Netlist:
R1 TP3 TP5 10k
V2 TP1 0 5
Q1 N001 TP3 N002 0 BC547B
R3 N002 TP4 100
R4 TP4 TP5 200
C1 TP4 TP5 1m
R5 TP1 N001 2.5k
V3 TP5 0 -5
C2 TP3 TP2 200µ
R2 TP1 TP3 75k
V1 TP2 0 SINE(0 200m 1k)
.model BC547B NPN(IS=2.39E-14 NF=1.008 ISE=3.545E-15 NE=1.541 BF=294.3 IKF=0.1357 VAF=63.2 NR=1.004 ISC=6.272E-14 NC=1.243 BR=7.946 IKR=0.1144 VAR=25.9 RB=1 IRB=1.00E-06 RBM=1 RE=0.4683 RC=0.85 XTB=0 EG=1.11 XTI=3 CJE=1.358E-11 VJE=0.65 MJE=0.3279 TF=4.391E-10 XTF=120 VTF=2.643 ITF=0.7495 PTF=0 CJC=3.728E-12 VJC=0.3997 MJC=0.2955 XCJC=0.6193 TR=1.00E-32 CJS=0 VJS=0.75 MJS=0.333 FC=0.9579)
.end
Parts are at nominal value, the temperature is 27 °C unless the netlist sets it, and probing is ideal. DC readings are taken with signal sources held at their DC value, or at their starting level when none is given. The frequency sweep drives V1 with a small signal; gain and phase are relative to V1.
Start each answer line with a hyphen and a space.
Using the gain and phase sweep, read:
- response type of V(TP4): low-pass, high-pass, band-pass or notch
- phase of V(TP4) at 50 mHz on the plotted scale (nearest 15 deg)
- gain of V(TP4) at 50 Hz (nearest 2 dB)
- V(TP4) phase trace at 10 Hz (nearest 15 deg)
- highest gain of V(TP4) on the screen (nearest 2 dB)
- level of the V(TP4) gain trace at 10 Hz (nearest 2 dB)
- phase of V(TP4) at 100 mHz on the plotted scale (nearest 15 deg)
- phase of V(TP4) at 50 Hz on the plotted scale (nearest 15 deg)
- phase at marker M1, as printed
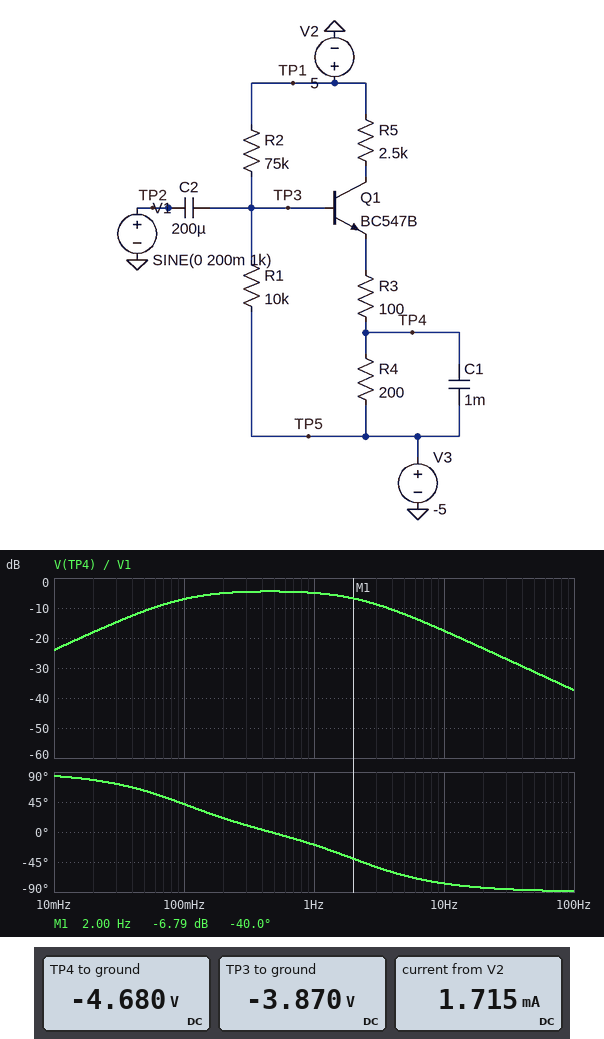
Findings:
- band-pass
- 60 deg
- -32 dB
- -75 deg
- -4 dB
- -18 dB
- 45 deg
- -90 deg
- -40.0 deg
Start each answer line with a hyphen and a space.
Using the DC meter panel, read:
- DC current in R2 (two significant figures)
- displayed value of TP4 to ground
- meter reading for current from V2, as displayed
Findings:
- 120 µA
- -4.680 V
- 1.715 mA
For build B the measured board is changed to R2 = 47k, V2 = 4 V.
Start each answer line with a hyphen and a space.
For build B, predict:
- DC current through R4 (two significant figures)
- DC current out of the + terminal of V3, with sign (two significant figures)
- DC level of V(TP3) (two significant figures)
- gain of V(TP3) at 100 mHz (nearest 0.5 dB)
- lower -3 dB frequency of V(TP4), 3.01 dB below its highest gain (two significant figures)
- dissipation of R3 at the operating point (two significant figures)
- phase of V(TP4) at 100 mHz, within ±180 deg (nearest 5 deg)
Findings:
- 2.8 mA
- -2.9 mA
- -3.5 V
- -3.5 dB
- 97 mHz
- 770 µW
- 45 deg
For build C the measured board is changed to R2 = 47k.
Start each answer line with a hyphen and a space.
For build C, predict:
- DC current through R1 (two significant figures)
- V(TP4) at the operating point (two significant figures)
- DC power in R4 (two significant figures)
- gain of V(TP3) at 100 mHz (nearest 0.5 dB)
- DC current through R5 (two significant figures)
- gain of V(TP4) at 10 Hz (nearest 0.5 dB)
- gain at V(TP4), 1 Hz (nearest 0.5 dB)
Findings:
- 170 µA
- -4.3 V
- 2.2 mW
- -3.5 dB
- 3.3 mA
- -17.0 dB
- -4.5 dB
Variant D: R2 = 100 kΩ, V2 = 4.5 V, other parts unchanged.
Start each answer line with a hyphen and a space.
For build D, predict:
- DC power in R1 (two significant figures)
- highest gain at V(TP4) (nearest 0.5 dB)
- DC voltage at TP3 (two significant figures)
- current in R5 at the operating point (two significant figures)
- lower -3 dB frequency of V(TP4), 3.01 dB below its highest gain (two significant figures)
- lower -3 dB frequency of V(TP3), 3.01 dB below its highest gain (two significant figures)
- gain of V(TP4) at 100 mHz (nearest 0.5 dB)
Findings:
- 71 µW
- -5.0 dB
- -4.2 V
- 720 µA
- 87 mHz
- 96 mHz
- -7.5 dB
